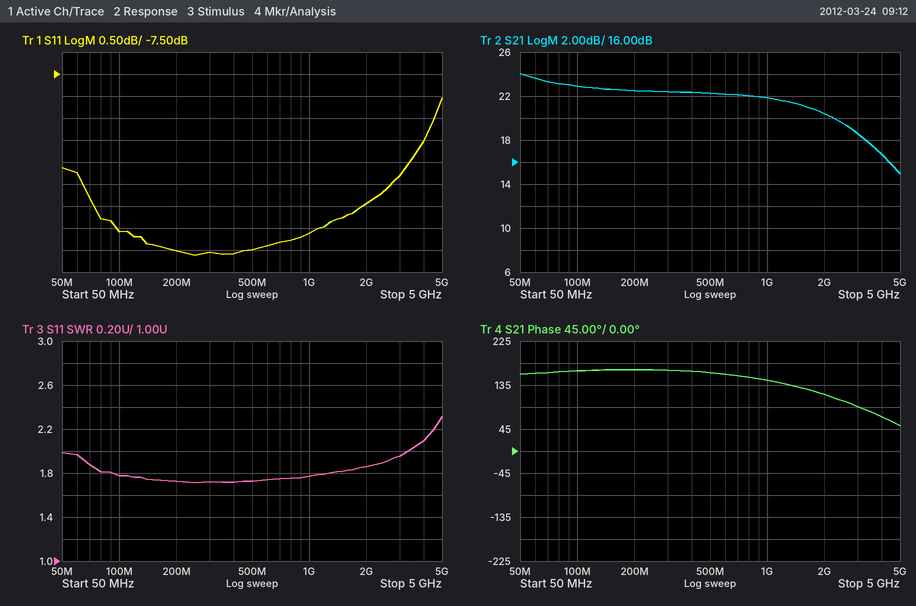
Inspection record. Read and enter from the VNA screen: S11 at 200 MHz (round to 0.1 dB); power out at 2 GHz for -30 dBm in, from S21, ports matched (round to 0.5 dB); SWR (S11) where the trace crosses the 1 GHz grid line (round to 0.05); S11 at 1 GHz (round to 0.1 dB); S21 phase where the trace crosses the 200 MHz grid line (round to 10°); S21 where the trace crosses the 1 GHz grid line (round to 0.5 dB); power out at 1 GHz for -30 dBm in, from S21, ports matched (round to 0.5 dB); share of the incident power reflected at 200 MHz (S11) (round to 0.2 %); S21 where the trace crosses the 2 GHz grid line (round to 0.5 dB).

-11.5 dB
-9.5 dBm
1.75
-11.1 dB
170°
22.0 dB
-8.0 dBm
7.0 %
20.5 dB
